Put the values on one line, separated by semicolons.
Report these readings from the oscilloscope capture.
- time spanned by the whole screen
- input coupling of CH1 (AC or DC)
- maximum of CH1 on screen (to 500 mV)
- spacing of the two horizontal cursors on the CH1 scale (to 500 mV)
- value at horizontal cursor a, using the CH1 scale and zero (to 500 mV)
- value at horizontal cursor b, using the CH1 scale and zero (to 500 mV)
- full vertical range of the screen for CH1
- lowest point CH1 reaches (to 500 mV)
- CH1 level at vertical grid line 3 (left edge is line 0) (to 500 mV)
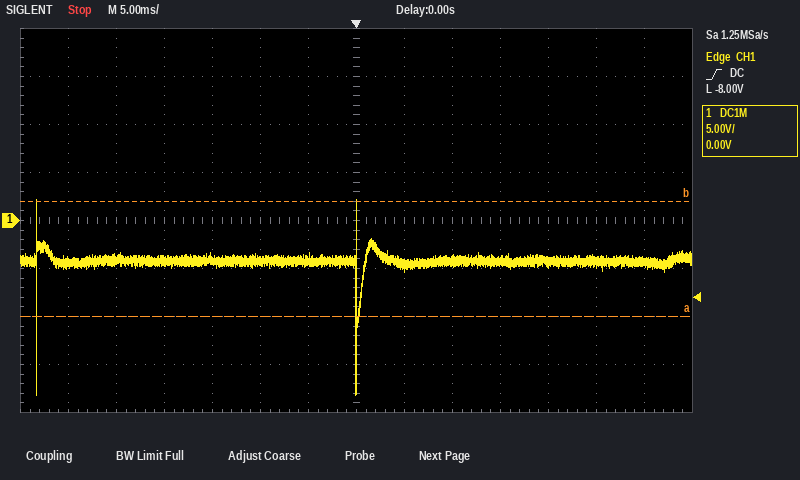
70 ms; DC; 2.0 V; 12.0 V; -10.0 V; 2.0 V; 40 V; -18.0 V; -4.0 V
